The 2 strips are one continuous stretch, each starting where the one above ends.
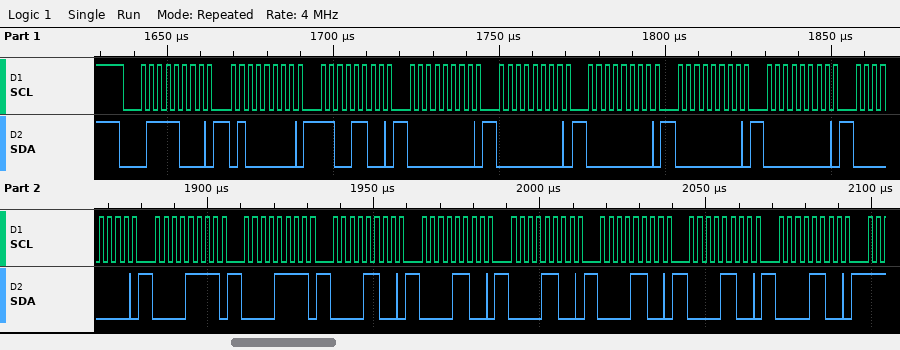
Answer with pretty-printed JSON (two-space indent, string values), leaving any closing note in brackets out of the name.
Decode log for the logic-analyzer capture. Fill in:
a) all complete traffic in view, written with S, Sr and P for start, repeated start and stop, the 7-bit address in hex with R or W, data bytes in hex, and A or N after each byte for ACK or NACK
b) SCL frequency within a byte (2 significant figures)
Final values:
{
  "all complete traffic in view, written with S, Sr and P for start, repeated start and stop, the 7-bit address in hex with R or W, data bytes in hex, and A or N after each byte for ACK or NACK": "S 3CW A 40 A CC A 00 A 00 A 00 A 00 A 00 A 00 A 0F A 0F A 0C A 0C A 0C A 0C A 0C A 0C A",
  "SCL frequency within a byte": "400 kHz"
}
